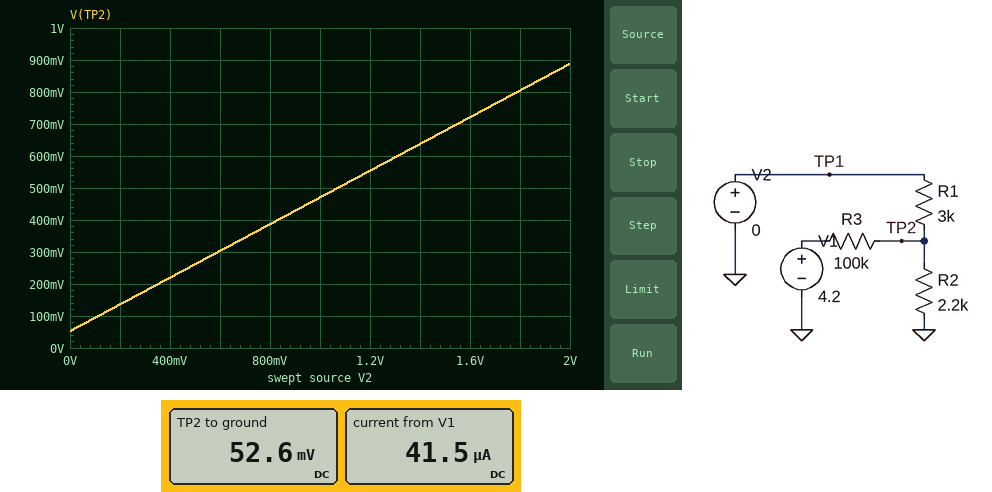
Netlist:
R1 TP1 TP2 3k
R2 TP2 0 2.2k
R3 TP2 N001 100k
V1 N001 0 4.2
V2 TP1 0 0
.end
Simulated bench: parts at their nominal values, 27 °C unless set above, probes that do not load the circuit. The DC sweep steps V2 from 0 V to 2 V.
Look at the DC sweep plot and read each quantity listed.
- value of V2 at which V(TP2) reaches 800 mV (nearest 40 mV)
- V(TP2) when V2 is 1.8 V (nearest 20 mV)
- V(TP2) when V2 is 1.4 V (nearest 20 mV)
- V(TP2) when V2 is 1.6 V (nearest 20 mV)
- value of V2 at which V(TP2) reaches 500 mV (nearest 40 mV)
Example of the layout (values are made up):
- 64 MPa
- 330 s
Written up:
- 1.80 V
- 800 mV
- 640 mV
- 720 mV
- 1.08 V
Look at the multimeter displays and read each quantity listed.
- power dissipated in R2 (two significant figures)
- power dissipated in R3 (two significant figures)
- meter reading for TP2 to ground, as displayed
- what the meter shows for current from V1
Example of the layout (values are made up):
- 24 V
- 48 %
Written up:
- 1.3 µW
- 170 µW
- 52.6 mV
- 41.5 µA
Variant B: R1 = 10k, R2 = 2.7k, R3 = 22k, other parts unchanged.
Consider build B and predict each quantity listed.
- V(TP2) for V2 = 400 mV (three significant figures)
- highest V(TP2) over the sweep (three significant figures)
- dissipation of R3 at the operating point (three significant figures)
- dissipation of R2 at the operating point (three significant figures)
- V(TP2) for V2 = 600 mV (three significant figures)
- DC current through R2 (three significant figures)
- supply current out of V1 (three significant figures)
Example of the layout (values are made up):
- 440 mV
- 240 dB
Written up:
- 448 mV
- 758 mV
- 667 µW
- 50.7 µW
- 486 mV
- 137 µA
- 174 µA
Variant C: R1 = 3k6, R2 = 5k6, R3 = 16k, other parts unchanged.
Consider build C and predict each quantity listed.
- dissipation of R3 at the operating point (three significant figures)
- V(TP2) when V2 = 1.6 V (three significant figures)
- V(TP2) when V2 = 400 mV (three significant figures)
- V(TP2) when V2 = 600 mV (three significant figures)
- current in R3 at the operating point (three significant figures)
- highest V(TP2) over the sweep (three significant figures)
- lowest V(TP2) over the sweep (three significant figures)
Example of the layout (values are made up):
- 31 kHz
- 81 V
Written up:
- 853 µW
- 1.36 V
- 720 mV
- 827 mV
- 231 µA
- 1.58 V
- 506 mV
